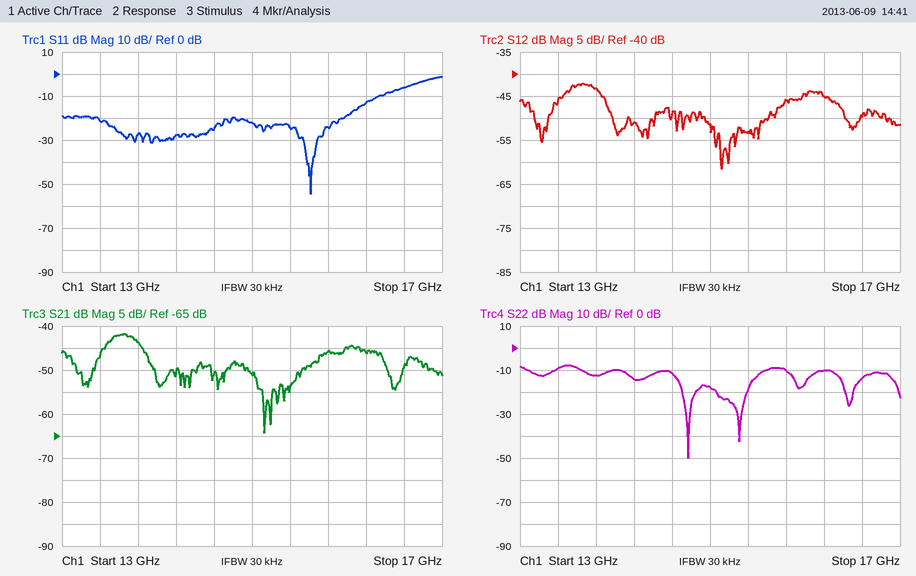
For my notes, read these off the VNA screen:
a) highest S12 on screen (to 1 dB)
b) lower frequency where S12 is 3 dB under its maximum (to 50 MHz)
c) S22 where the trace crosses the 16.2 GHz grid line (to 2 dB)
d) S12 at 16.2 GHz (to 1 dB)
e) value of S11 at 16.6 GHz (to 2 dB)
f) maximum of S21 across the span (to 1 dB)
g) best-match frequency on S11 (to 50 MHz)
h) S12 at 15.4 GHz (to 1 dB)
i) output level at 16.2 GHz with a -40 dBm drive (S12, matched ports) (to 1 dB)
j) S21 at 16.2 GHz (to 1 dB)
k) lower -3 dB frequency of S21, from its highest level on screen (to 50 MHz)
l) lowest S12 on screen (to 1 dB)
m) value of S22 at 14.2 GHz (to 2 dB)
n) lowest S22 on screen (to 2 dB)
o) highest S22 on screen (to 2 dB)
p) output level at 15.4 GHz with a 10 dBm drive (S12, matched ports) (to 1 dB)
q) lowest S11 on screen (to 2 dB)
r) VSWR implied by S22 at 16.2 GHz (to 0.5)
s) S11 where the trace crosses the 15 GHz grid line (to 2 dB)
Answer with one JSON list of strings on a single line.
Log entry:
["-42 dB", "13.45 GHz", "-10 dB", "-45 dB", "-6 dB", "-42 dB", "15.60 GHz", "-53 dB", "-85 dBm", "-46 dB", "13.45 GHz", "-62 dB", "-14 dB", "-50 dB", "-8 dB", "-43 dBm", "-54 dB", "2.0", "-22 dB"]
